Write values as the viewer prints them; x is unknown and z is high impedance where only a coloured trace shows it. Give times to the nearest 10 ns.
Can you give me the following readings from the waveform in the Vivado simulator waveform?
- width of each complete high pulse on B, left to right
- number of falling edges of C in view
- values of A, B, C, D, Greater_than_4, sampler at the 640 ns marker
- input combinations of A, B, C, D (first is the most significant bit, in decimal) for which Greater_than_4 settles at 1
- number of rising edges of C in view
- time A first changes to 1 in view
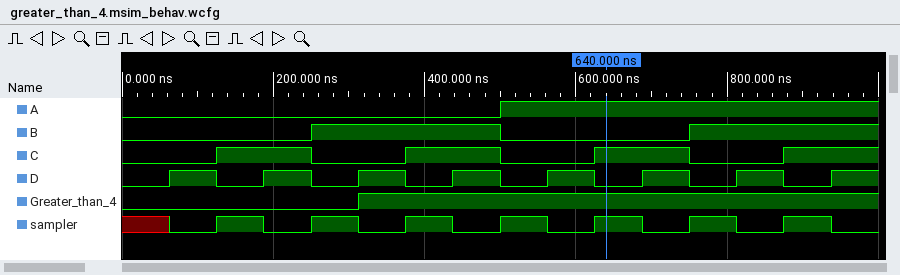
250 ns
3
A=1, B=0, C=1, D=0, Greater_than_4=1, sampler=1
5, 6, 7, 8, 9, 10, 11, 12, 13, 14, 15
4
500 ns
